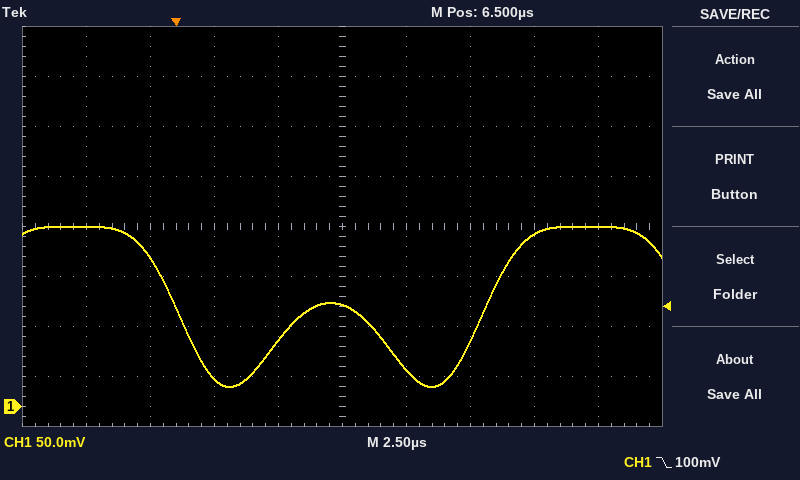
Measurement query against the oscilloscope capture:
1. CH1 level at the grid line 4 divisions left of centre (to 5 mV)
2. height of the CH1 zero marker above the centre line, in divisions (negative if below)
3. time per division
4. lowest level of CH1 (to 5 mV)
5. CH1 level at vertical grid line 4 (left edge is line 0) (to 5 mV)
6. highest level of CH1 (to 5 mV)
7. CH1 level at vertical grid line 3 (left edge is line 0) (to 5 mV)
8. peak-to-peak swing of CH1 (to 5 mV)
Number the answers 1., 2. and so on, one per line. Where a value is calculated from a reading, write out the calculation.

1. 180 mV
2. -3.6 div
3. 2.5 µs
4. 20 mV
5. 65 mV
6. 180 mV
7. 30 mV
8. 180 mV − (20 mV) = 160 mV
